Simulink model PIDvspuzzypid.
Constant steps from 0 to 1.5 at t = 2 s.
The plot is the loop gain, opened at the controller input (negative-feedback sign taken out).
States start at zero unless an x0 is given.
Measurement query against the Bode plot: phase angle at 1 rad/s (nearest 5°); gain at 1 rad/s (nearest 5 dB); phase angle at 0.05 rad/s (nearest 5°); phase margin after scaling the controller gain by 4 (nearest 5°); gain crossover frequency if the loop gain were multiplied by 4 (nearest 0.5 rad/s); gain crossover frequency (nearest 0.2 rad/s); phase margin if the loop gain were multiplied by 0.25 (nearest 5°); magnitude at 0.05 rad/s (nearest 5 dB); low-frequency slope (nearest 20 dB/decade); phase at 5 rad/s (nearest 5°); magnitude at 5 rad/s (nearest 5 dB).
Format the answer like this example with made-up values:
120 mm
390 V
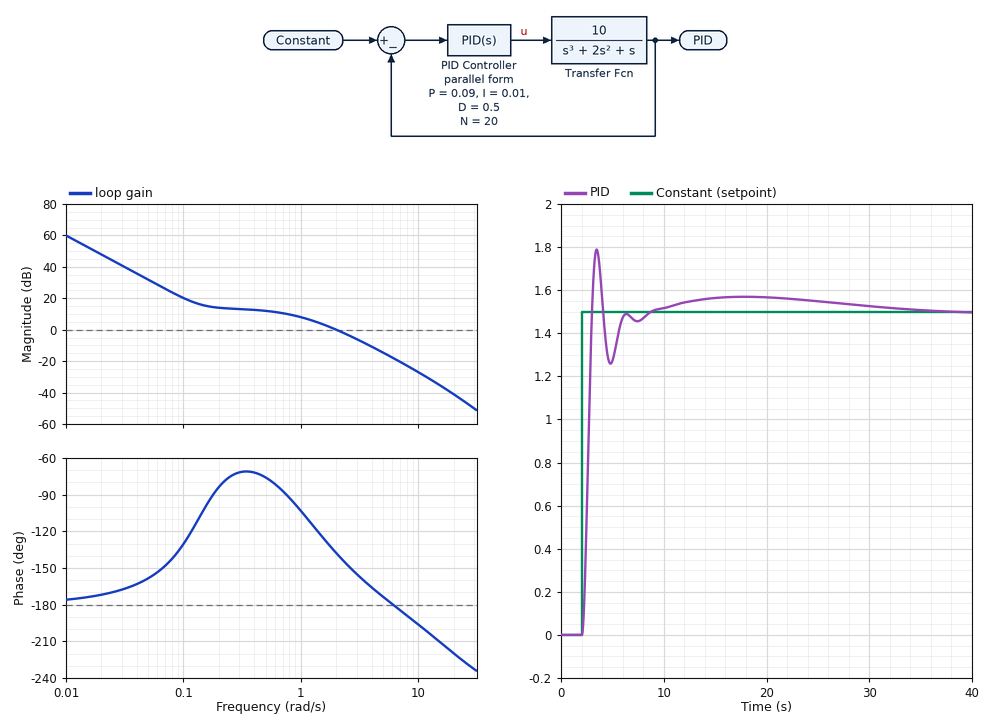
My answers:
-105°
10 dB
-160°
10°
4.5 rad/s
2.0 rad/s
105°
30 dB
-40 dB/decade
-175°
-15 dB
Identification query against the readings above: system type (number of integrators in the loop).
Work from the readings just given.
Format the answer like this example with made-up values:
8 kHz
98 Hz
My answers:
2
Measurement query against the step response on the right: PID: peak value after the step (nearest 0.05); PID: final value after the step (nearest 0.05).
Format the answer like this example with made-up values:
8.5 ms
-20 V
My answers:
1.80
1.50
